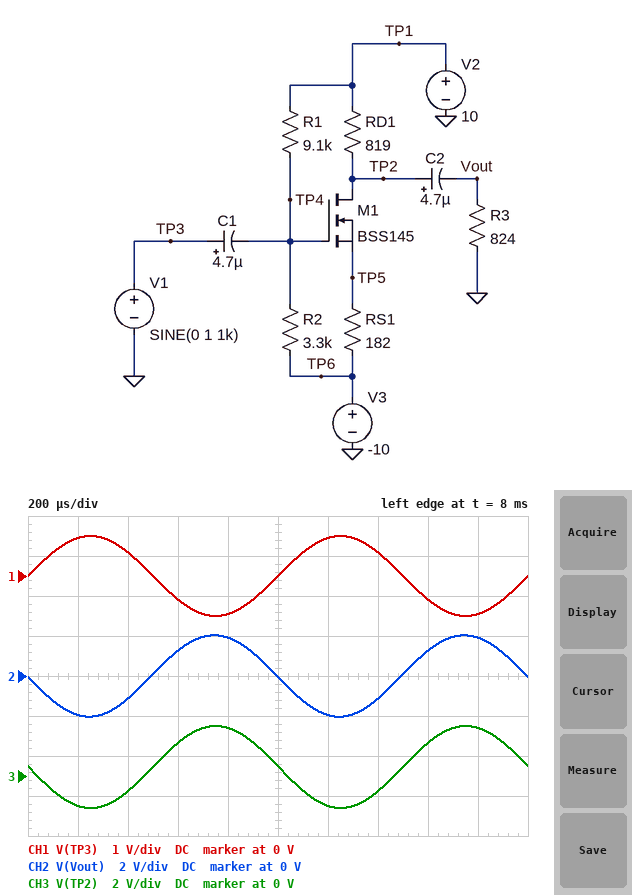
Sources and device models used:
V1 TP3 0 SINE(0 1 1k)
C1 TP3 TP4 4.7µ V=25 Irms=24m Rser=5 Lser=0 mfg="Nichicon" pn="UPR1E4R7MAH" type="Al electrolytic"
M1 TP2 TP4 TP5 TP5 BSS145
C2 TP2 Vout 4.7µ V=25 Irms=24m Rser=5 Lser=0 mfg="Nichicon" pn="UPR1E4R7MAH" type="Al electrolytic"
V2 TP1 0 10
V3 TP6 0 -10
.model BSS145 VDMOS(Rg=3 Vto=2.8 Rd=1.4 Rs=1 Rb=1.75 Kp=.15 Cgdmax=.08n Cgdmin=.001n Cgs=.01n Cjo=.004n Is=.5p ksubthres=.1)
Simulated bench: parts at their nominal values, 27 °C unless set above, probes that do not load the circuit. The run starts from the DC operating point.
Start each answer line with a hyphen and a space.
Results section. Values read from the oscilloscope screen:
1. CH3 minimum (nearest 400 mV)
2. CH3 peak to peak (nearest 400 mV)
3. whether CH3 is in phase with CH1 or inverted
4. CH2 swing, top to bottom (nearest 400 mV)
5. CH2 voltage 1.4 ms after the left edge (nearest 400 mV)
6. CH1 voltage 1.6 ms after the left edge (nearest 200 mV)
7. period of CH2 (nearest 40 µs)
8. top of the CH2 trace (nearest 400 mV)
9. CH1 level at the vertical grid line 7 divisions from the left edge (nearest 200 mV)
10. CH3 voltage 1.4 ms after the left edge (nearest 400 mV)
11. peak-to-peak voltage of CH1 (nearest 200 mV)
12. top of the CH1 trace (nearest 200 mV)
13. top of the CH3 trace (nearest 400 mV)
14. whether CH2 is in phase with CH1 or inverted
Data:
- -1.6 V
- 4.0 V
- inverted
- 4.0 V
- -1.2 V
- -600 mV
- 1.00 ms
- 2.0 V
- 600 mV
- -800 mV
- 2.0 V
- 1.0 V
- 2.4 V
- inverted
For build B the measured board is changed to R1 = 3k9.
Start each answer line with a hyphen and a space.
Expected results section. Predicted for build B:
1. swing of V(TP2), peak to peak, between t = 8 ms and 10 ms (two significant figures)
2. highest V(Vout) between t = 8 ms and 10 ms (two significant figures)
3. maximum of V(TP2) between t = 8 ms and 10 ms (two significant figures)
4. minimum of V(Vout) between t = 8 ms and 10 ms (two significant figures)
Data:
- 29 mV
- 18 mV
- -6.3 V
- -11 mV
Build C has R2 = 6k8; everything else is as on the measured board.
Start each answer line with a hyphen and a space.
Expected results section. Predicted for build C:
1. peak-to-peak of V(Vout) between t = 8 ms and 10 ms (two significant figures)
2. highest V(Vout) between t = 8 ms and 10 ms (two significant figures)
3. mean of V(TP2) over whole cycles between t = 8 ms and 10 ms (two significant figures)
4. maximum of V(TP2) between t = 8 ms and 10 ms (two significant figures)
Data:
- 55 mV
- 36 mV
- -6.3 V
- -6.2 V
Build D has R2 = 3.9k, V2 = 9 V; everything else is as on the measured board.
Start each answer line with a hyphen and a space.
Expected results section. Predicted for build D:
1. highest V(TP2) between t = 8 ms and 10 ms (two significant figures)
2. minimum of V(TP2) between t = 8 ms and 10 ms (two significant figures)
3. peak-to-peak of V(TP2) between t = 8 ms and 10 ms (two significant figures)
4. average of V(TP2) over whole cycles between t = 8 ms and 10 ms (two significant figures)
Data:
- -30 mV
- -4.2 V
- 4.1 V
- -2.1 V
